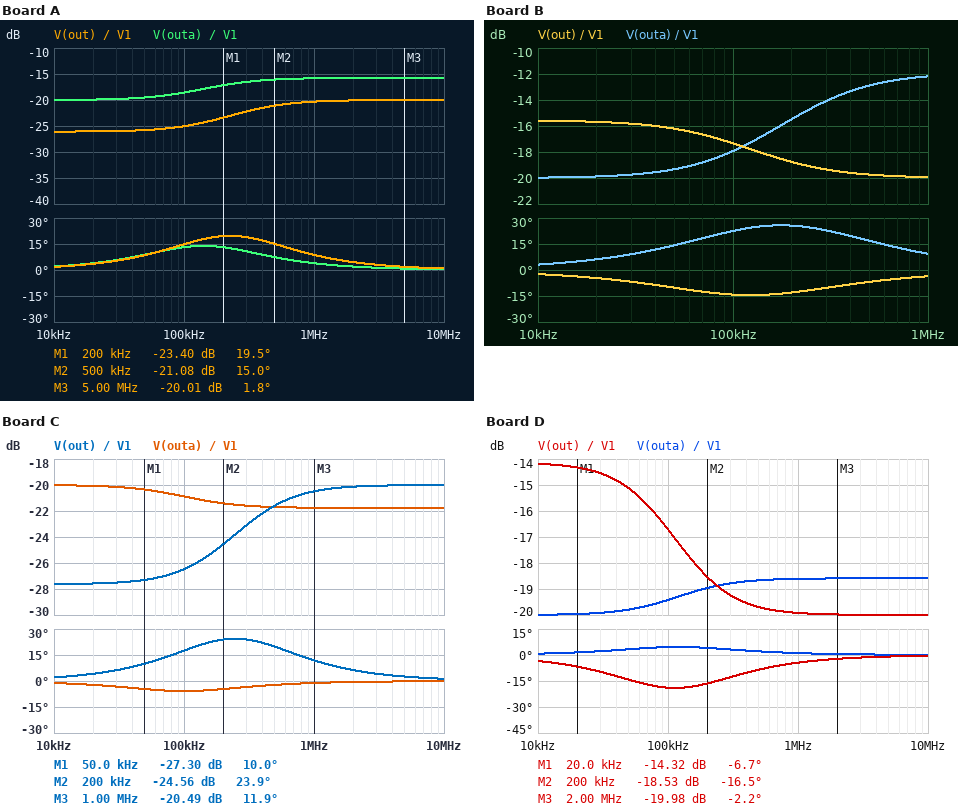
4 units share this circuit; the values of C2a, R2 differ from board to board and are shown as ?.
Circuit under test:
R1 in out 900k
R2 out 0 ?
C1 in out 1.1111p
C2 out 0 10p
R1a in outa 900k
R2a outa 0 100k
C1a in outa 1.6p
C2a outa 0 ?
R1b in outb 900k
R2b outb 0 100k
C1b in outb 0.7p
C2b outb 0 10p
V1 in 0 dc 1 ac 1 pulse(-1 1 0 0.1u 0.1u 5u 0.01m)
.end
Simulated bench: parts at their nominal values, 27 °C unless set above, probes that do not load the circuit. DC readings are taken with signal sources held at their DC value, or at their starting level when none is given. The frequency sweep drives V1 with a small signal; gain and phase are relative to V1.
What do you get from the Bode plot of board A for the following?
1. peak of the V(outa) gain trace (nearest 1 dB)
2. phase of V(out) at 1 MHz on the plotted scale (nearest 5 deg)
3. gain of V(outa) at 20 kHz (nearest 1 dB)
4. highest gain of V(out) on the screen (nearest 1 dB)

-16 dB
10 deg
-20 dB
-20 dB
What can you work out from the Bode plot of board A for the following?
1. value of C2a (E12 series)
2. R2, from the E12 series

8.2 pF
47 kΩ
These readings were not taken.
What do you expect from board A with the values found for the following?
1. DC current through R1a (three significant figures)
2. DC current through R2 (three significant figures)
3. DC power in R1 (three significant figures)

1.00 µA
1.06 µA
1.00 µW
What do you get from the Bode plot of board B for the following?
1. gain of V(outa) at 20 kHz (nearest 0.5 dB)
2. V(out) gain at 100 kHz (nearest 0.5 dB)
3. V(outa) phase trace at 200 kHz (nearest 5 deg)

-20.0 dB
-17.5 dB
25 deg
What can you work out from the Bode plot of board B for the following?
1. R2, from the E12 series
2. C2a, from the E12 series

180 kΩ
4.7 pF
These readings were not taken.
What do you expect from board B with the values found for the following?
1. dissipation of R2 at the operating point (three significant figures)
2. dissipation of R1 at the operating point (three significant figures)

154 nW
772 nW
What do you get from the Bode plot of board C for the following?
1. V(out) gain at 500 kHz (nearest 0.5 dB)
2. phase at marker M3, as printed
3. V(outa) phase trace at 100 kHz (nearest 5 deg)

-21.5 dB
11.9 deg
-5 deg
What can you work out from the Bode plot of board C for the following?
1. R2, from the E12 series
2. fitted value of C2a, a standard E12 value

39 kΩ
18 pF
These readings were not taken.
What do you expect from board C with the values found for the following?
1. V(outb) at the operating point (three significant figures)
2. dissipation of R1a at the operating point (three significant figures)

100 mV
900 nW
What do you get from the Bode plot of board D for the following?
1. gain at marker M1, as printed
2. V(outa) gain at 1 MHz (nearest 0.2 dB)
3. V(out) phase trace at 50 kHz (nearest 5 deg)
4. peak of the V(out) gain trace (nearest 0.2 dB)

-14.32 dB
-18.6 dB
-15 deg
-14.2 dB
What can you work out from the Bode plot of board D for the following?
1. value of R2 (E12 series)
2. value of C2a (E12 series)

220 kΩ
12 pF
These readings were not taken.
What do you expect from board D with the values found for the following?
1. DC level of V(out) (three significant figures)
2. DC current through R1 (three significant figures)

196 mV
893 nA
